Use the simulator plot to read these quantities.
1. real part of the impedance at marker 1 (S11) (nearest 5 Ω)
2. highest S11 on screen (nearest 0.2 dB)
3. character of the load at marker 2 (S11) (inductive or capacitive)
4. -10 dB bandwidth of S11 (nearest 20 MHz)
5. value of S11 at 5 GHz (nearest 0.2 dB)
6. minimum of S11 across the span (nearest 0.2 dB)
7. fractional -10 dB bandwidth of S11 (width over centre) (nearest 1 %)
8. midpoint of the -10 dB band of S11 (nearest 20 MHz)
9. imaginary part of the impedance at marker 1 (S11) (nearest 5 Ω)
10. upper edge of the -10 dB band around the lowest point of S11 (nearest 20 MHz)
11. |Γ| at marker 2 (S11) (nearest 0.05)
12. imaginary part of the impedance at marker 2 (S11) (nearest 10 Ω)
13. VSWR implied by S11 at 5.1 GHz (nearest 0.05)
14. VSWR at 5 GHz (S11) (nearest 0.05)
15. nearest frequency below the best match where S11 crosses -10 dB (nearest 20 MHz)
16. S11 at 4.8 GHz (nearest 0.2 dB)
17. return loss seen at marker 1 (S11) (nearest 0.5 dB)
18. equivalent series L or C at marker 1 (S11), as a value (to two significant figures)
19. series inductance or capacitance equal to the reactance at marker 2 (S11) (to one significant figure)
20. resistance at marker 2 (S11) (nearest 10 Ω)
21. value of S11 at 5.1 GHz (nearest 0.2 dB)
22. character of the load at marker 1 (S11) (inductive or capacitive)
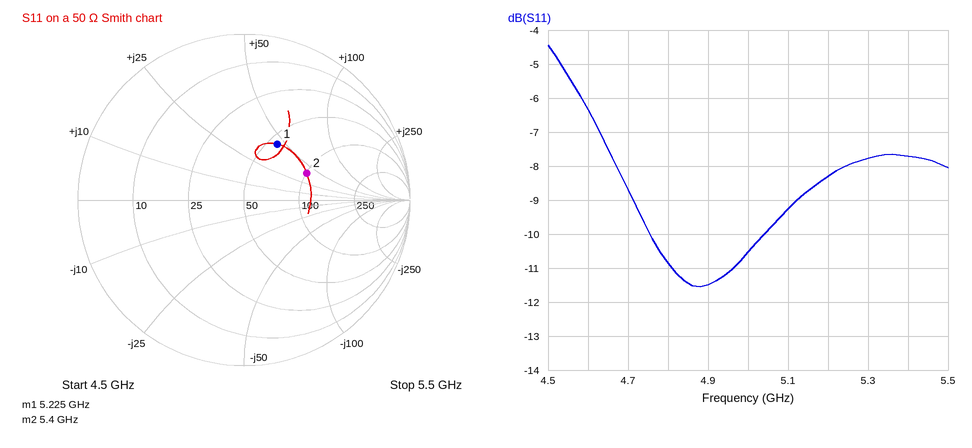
55 Ω
-4.4 dB
inductive
280 MHz
-10.6 dB
-11.6 dB
6 %
4.90 GHz
+45 Ω
5.04 GHz
0.40
+40 Ω
2.05
1.85
4.76 GHz
-10.8 dB
8.0 dB
1.4 nH
1 nH
100 Ω
-9.2 dB
inductive
